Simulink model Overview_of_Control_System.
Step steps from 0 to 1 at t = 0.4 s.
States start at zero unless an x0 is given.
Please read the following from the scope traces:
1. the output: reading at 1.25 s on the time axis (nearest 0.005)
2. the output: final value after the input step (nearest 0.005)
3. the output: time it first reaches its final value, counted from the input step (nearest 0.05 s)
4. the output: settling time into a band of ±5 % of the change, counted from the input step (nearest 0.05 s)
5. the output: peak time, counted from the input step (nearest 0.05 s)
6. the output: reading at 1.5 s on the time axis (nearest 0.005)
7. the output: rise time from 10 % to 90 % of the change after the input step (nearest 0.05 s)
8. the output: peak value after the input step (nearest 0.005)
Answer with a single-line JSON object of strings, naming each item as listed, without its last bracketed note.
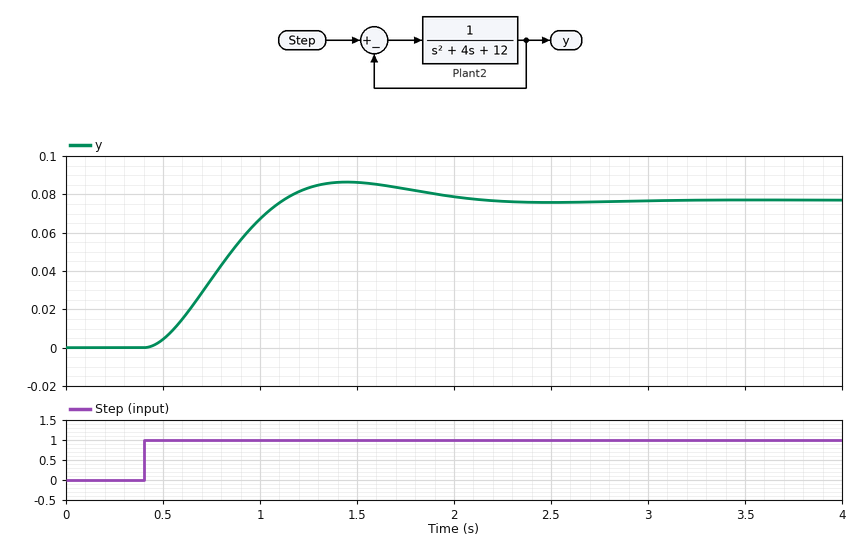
{"the output: reading at 1.25 s on the time axis": "0.085", "the output: final value after the input step": "0.075", "the output: time it first reaches its final value, counted from the input step": "0.70 s", "the output: settling time into a band of ±5 % of the change, counted from the input step": "1.45 s", "the output: peak time, counted from the input step": "1.05 s", "the output: reading at 1.5 s on the time axis": "0.085", "the output: rise time from 10 % to 90 % of the change after the input step": "0.50 s", "the output: peak value after the input step": "0.085"}
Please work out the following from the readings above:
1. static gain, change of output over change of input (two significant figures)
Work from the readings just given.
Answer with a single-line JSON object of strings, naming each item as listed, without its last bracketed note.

{"static gain, change of output over change of input": "0.075"}
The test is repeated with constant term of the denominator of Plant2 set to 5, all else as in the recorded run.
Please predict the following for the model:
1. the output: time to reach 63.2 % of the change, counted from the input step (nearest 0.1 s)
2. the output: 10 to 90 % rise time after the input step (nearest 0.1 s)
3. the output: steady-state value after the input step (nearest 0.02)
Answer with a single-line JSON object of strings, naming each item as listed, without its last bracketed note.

{"the output: time to reach 63.2 % of the change, counted from the input step": "0.8 s", "the output: 10 to 90 % rise time after the input step": "1.0 s", "the output: steady-state value after the input step": "0.16"}
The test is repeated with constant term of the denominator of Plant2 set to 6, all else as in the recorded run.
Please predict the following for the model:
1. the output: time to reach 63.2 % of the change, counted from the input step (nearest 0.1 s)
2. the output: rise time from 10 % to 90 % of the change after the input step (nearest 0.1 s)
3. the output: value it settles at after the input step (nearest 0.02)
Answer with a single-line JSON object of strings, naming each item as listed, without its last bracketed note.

{"the output: time to reach 63.2 % of the change, counted from the input step": "0.7 s", "the output: rise time from 10 % to 90 % of the change after the input step": "0.9 s", "the output: value it settles at after the input step": "0.14"}
